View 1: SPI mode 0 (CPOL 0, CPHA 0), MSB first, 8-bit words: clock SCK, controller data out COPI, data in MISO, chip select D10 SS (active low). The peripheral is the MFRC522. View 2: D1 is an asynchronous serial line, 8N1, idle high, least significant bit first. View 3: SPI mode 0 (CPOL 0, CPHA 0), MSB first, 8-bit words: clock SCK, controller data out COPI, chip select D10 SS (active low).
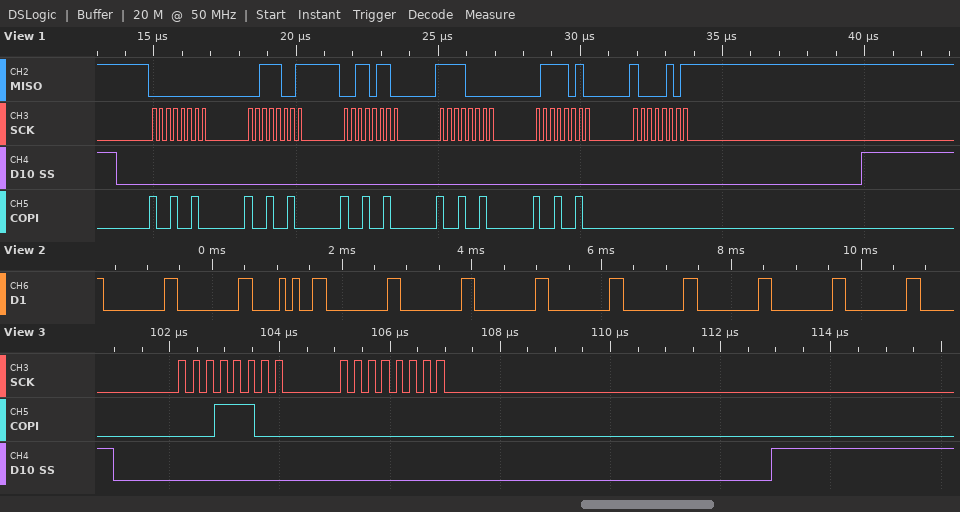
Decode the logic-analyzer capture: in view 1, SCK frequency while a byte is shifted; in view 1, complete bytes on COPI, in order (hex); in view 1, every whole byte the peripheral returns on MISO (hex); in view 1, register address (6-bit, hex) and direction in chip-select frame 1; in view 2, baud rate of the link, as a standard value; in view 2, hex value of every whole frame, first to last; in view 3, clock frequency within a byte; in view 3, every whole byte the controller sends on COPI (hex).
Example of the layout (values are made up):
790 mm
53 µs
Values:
4 MHz
92 92 92 92 92 00
00 39 36 F0 7A 85
0x09 read
9600 baud
00 00 28 00 00 00 00 00 00 00 00
4 MHz
1C 00
